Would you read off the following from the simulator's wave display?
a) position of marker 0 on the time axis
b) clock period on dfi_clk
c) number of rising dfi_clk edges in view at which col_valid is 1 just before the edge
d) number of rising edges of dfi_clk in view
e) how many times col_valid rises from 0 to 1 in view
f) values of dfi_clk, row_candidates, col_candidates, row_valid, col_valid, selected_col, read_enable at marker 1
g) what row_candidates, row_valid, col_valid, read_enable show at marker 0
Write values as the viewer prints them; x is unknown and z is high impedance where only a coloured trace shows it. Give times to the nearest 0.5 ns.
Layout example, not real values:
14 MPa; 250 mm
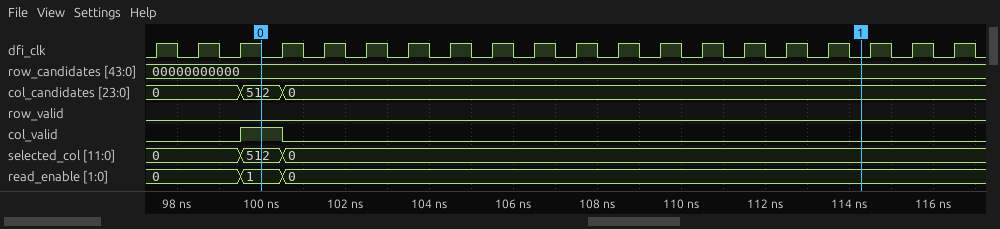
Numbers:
100 ns; 1 ns; 1; 20; 1; dfi_clk=0, row_candidates=00000000000, col_candidates=0, row_valid=0, col_valid=0, selected_col=0, read_enable=0; row_candidates=00000000000, row_valid=0, col_valid=1, read_enable=1
